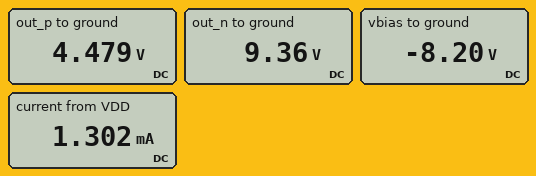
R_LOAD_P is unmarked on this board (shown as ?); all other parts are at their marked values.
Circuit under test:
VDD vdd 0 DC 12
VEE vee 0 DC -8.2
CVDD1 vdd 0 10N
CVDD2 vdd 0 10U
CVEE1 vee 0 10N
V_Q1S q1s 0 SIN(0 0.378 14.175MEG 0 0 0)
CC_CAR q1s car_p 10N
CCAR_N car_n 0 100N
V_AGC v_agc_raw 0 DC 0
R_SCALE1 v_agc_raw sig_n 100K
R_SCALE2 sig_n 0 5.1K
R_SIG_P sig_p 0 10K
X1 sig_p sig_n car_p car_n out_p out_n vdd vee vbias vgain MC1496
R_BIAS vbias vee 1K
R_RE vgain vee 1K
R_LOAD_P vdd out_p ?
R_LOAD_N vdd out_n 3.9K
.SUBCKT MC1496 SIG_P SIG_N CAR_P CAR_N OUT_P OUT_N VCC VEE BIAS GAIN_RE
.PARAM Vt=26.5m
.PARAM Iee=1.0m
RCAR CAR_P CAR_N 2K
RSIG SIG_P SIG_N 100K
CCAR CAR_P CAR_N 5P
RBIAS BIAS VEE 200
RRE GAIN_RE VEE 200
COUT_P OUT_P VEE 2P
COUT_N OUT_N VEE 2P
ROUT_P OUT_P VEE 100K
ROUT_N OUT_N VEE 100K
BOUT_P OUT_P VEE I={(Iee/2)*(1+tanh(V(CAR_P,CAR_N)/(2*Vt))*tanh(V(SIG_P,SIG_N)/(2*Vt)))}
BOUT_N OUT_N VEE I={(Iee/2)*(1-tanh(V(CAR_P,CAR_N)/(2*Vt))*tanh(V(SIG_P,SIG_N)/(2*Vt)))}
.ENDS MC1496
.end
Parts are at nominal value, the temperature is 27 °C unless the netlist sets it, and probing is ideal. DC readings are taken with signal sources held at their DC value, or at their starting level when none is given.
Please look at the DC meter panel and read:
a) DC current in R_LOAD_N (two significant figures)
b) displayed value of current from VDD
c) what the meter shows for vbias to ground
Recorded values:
680 µA
1.302 mA
-8.20 V
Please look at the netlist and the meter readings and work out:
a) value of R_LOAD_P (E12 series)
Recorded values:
12 kΩ
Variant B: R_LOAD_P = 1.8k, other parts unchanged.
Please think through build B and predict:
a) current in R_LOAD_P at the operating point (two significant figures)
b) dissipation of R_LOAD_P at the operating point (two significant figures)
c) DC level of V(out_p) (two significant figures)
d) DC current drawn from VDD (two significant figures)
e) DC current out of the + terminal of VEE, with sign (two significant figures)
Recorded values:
690 µA
860 µW
11 V
1.4 mA
-1.4 mA
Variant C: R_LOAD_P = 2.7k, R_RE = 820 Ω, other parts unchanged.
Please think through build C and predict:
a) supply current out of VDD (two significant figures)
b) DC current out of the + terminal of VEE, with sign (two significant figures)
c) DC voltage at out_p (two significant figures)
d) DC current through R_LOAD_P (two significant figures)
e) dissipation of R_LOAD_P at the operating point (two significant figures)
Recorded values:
1.4 mA
-1.4 mA
10 V
680 µA
1.3 mW
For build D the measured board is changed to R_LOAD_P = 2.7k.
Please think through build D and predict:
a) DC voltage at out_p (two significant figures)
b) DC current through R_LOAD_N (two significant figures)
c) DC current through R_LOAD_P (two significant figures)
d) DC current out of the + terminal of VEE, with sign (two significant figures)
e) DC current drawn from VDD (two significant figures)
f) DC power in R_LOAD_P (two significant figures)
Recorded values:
10 V
680 µA
680 µA
-1.4 mA
1.4 mA
1.3 mW
